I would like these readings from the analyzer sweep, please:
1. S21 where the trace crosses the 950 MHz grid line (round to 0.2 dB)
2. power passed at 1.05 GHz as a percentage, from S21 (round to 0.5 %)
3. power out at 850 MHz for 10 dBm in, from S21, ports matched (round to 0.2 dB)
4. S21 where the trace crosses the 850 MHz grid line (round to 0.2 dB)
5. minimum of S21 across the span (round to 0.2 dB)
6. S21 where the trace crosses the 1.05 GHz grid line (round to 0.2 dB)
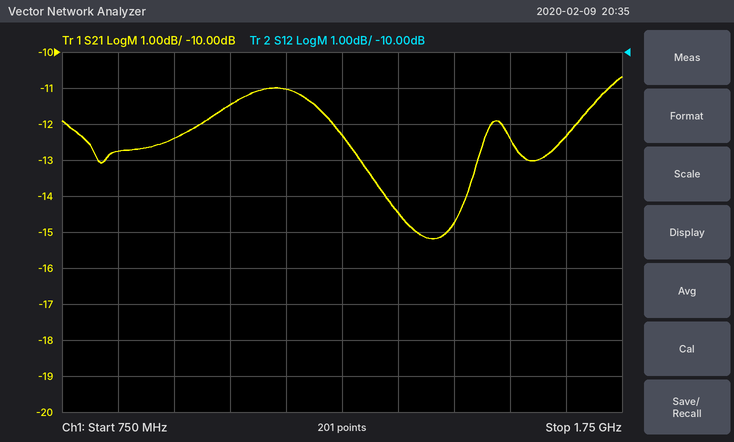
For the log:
-12.4 dB
7.0 %
-2.8 dBm
-12.8 dB
-15.2 dB
-11.4 dB
